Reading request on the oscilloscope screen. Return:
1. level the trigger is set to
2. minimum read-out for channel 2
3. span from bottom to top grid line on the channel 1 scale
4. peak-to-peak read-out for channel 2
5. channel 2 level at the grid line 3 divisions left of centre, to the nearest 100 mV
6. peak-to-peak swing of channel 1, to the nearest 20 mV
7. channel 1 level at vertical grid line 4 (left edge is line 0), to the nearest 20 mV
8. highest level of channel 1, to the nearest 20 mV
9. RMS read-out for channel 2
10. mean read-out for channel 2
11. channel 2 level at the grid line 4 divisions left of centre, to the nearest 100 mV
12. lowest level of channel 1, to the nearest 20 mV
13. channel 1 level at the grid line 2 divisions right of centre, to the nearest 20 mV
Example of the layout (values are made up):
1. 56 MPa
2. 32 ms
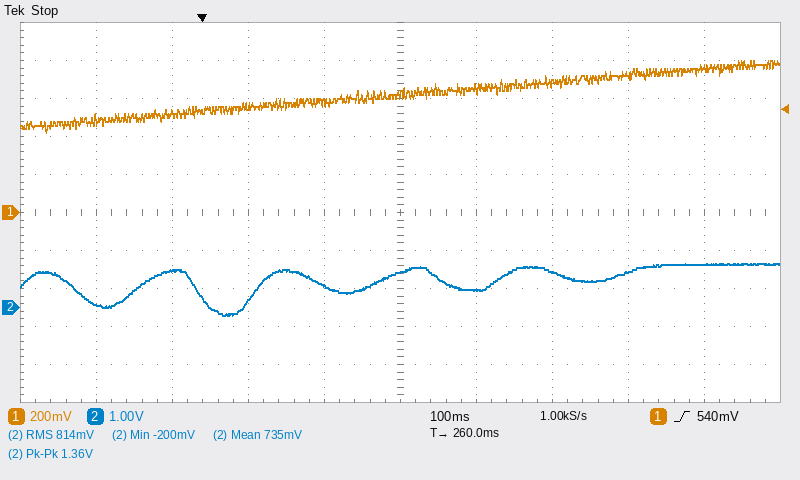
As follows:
1. 540 mV
2. -200 mV
3. 2 V
4. 1.36 V
5. 1.0 V
6. 380 mV
7. 580 mV
8. 800 mV
9. 814 mV
10. 735 mV
11. 100 mV
12. 420 mV
13. 680 mV
